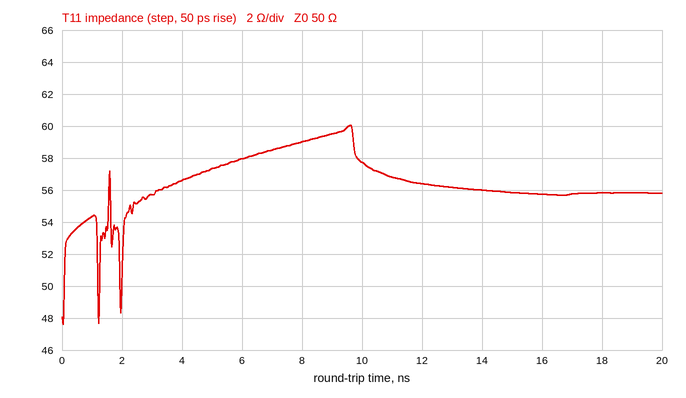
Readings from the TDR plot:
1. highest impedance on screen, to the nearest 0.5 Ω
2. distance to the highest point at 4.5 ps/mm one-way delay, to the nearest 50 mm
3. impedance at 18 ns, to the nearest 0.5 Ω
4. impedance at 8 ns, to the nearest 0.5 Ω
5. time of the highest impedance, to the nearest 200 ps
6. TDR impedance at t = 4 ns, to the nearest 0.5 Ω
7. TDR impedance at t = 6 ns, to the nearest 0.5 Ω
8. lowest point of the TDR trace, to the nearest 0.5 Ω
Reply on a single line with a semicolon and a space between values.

60.0 Ω; 1.05 m; 56.0 Ω; 59.0 Ω; 9.6 ns; 56.5 Ω; 58.0 Ω; 47.5 Ω
